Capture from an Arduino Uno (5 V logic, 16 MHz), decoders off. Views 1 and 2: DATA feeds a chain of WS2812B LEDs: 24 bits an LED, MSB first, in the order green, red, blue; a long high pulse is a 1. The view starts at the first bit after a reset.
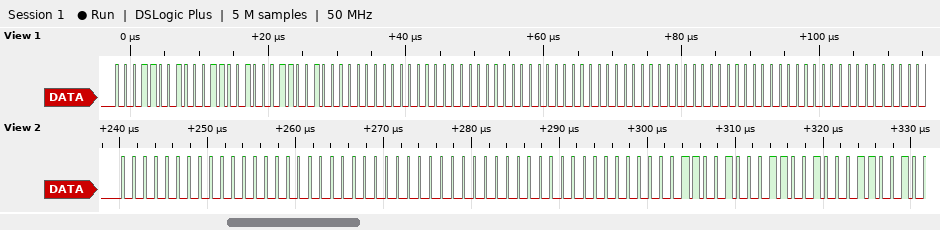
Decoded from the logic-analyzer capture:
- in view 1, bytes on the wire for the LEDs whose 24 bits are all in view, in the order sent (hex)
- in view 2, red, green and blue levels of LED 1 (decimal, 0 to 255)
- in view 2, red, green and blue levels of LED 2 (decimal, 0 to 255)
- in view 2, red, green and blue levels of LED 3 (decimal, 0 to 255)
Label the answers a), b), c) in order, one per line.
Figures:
a) 19 19 19 00 00 00 00 00 00
b) 0, 0, 0
c) 0, 0, 0
d) 25, 25, 25
